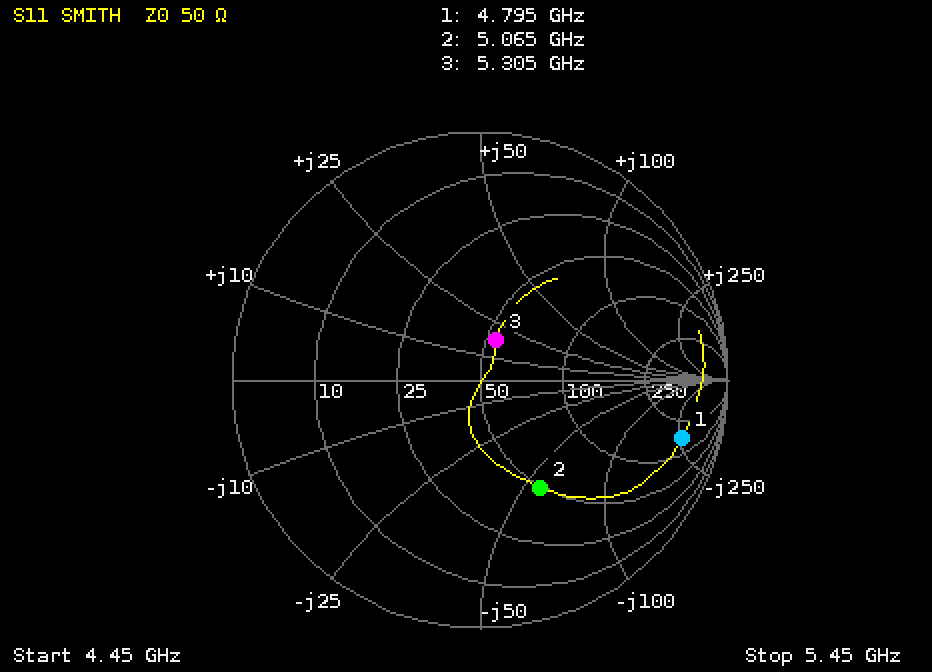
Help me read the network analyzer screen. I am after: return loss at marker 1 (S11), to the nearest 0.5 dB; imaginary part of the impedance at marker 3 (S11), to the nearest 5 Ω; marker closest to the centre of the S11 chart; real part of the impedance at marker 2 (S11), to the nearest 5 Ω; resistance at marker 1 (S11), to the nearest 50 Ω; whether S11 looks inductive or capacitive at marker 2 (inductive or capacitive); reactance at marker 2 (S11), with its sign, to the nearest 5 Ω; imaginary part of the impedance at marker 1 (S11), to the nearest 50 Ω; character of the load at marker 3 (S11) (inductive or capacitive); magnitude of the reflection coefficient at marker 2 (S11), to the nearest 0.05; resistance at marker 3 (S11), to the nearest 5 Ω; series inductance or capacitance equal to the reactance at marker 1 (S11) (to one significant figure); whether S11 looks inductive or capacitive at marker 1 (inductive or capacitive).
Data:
1.5 dB
+20 Ω
marker 3
50 Ω
150 Ω
capacitive
-55 Ω
-250 Ω
inductive
0.50
55 Ω
100 fF
capacitive
